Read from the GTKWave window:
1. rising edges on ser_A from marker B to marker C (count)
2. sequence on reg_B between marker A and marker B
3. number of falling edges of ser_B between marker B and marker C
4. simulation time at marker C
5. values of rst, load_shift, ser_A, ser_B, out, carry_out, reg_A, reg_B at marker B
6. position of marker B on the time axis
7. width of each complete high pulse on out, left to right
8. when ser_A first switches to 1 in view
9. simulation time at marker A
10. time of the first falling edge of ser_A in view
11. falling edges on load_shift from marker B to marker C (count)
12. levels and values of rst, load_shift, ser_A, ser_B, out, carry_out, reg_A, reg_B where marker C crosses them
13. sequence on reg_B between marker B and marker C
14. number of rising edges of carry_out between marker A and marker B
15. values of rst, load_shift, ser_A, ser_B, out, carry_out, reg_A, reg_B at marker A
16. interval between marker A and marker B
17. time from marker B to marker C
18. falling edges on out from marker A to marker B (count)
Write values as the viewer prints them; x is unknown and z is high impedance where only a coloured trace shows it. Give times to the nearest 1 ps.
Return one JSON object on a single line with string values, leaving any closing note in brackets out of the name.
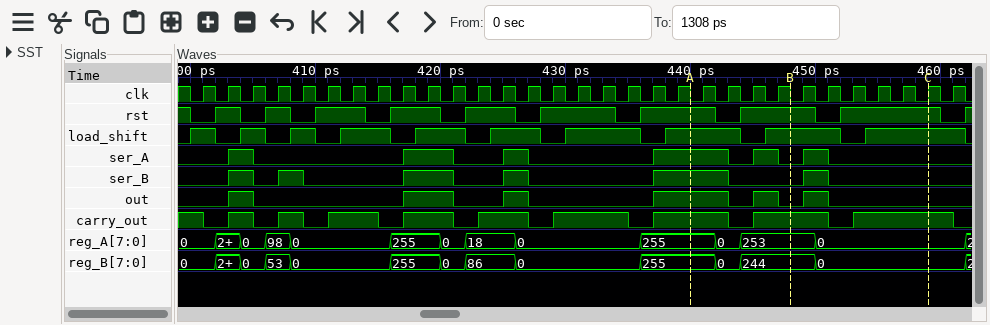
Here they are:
{"rising edges on ser_A from marker B to marker C": "1", "sequence on reg_B between marker A and marker B": "255, 0, 244", "number of falling edges of ser_B between marker B and marker C": "1", "simulation time at marker C": "459 ps", "values of rst, load_shift, ser_A, ser_B, out, carry_out, reg_A, reg_B at marker B": "rst=1, load_shift=1, ser_A=0, ser_B=0, out=0, carry_out=1, reg_A=253, reg_B=244", "position of marker B on the time axis": "448 ps", "width of each complete high pulse on out, left to right": "2 ps, 4 ps, 2 ps, 6 ps, 2 ps, 2 ps", "when ser_A first switches to 1 in view": "403 ps", "simulation time at marker A": "440 ps", "time of the first falling edge of ser_A in view": "405 ps", "falling edges on load_shift from marker B to marker C": "1", "levels and values of rst, load_shift, ser_A, ser_B, out, carry_out, reg_A, reg_B where marker C crosses them": "rst=1, load_shift=1, ser_A=0, ser_B=0, out=0, carry_out=1, reg_A=0, reg_B=0", "sequence on reg_B between marker B and marker C": "244, 0", "number of rising edges of carry_out between marker A and marker B": "1", "values of rst, load_shift, ser_A, ser_B, out, carry_out, reg_A, reg_B at marker A": "rst=1, load_shift=1, ser_A=1, ser_B=1, out=1, carry_out=1, reg_A=255, reg_B=255", "interval between marker A and marker B": "8 ps", "time from marker B to marker C": "11 ps", "falling edges on out from marker A to marker B": "2"}
